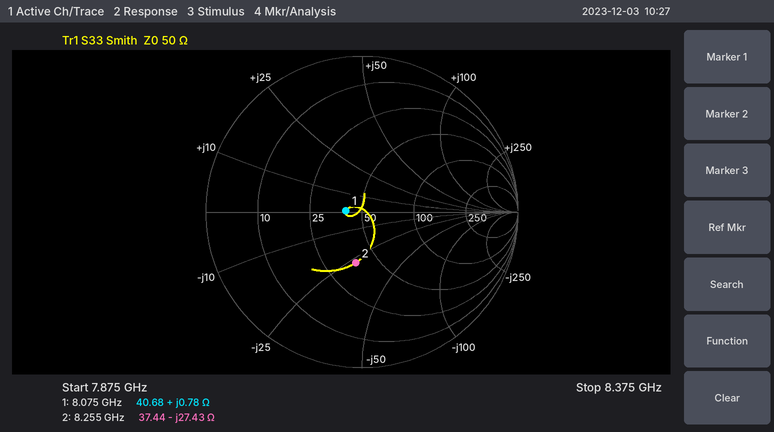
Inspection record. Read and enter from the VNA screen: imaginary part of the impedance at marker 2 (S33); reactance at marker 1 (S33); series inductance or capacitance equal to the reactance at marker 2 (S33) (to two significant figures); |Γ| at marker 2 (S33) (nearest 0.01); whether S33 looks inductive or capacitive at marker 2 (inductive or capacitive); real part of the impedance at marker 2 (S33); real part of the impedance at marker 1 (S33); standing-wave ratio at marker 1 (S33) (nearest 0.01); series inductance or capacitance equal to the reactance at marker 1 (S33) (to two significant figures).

-27.43 Ω
+0.78 Ω
700 fF
0.33
capacitive
37.44 Ω
40.68 Ω
1.23
15 pH
